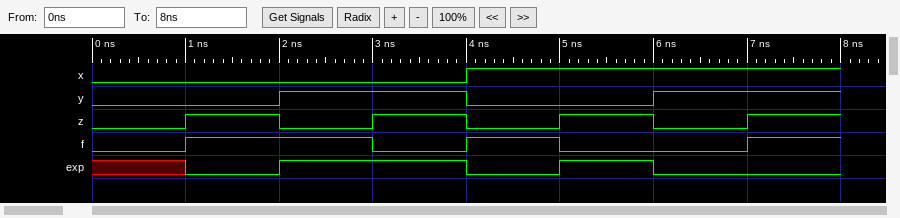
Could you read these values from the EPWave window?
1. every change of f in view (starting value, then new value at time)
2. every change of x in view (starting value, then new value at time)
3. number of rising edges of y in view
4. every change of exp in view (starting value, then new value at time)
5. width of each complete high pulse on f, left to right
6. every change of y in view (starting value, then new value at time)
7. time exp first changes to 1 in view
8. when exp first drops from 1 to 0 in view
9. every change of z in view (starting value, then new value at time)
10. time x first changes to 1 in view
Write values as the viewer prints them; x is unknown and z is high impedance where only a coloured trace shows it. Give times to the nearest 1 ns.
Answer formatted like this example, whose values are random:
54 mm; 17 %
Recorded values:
0, 1 at 1 ns, 0 at 3 ns, 1 at 4 ns, 0 at 5 ns, 1 at 7 ns; 0, 1 at 4 ns; 2; x, 0 at 1 ns, 1 at 2 ns, 0 at 4 ns, 1 at 5 ns, 0 at 6 ns; 2 ns, 1 ns; 0, 1 at 2 ns, 0 at 4 ns, 1 at 6 ns; 2 ns; 4 ns; 0, 1 at 1 ns, 0 at 2 ns, 1 at 3 ns, 0 at 4 ns, 1 at 5 ns, 0 at 6 ns, 1 at 7 ns; 4 ns
